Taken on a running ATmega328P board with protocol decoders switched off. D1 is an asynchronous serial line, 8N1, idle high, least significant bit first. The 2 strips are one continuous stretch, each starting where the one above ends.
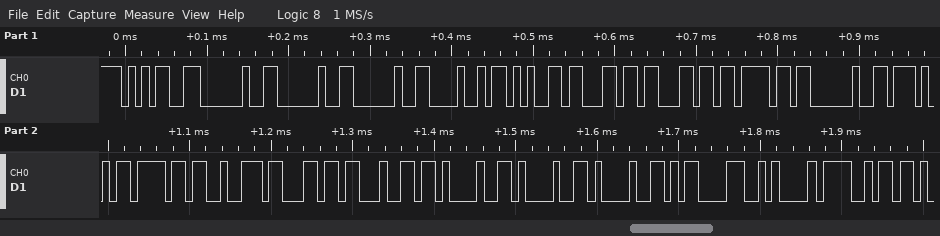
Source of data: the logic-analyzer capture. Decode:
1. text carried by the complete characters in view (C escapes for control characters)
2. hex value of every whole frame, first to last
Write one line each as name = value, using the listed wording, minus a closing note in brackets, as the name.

text carried by the complete characters in view = "5   Hello World!!!\r\nO"
hex value of every whole frame, first to last = 35 20 20 20 48 65 6C 6C 6F 20 57 6F 72 6C 64 21 21 21 0D 0A 4F
